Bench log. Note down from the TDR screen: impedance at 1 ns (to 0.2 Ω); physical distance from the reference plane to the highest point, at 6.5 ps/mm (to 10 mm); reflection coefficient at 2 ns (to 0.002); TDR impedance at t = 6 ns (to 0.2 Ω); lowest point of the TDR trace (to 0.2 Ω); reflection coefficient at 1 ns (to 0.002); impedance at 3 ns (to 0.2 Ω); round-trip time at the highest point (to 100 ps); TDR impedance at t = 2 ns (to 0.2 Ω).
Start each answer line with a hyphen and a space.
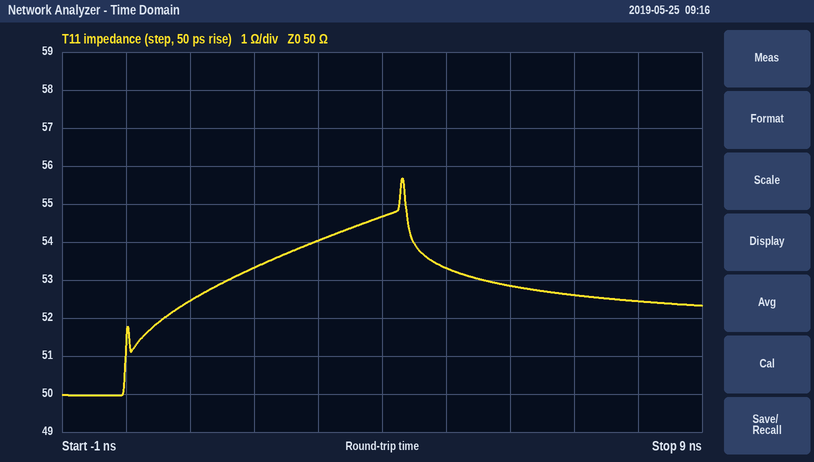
- 52.4 Ω
- 330 mm
- +0.032
- 52.8 Ω
- 50.0 Ω
- +0.024
- 54.0 Ω
- 4.3 ns
- 53.4 Ω
